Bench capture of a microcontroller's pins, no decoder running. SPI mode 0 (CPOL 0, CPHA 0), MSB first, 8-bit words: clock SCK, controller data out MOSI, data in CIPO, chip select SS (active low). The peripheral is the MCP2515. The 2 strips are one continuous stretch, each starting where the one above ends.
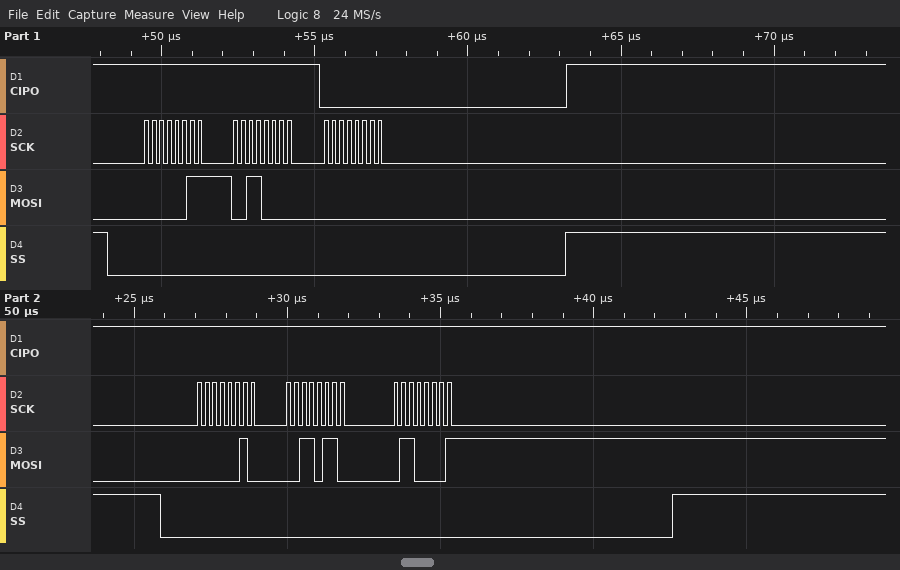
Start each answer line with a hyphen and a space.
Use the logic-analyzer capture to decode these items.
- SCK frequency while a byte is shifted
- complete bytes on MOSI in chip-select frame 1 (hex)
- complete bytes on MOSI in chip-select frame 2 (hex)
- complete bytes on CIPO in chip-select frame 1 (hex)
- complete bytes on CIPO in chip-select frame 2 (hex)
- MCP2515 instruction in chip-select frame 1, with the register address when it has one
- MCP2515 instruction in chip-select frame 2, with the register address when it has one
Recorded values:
- 4 MHz
- 03 30 00
- 02 36 61
- FF FF 00
- FF FF FF
- READ 0x30
- WRITE 0x36
